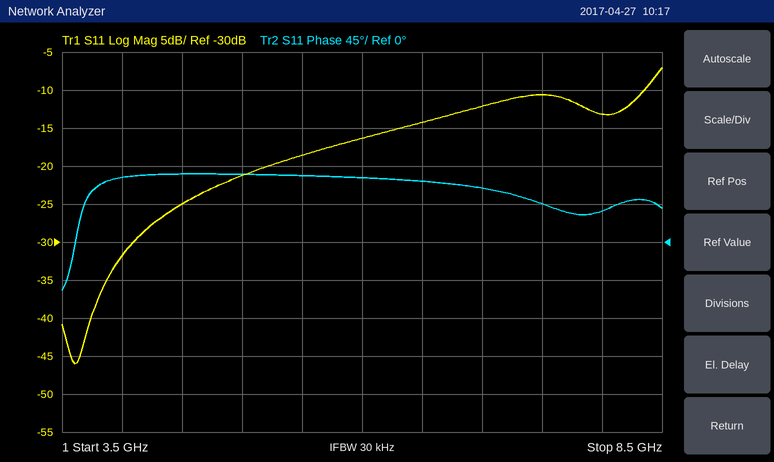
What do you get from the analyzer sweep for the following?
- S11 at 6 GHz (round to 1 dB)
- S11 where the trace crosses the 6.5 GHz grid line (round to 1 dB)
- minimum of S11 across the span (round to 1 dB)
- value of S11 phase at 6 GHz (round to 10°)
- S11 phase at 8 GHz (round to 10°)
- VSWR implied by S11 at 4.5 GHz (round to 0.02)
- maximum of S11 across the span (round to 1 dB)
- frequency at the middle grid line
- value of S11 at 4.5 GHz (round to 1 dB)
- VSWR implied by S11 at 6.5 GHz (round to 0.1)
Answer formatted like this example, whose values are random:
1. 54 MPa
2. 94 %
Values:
1. -16 dB
2. -14 dB
3. -46 dB
4. 80°
5. 40°
6. 1.12
7. -7 dB
8. 6 GHz
9. -25 dB
10. 1.5
